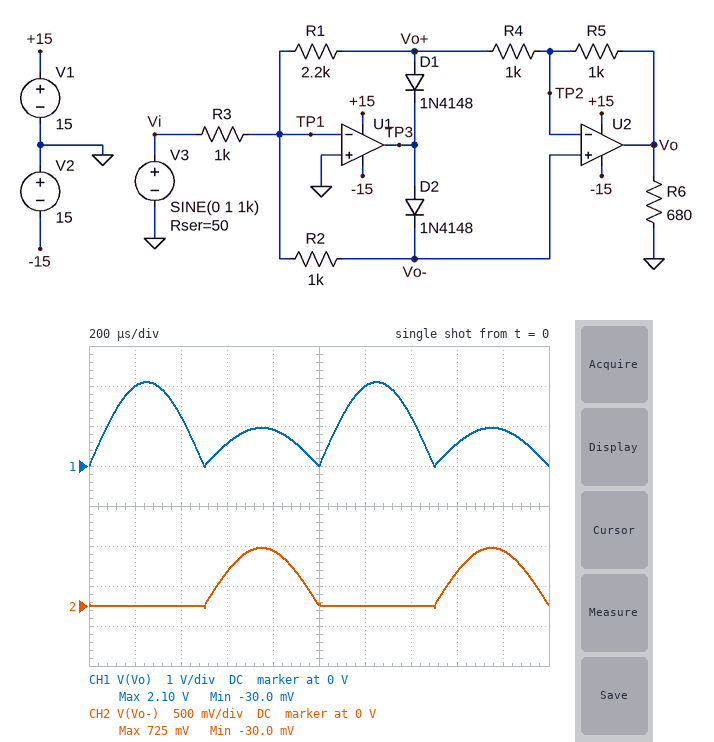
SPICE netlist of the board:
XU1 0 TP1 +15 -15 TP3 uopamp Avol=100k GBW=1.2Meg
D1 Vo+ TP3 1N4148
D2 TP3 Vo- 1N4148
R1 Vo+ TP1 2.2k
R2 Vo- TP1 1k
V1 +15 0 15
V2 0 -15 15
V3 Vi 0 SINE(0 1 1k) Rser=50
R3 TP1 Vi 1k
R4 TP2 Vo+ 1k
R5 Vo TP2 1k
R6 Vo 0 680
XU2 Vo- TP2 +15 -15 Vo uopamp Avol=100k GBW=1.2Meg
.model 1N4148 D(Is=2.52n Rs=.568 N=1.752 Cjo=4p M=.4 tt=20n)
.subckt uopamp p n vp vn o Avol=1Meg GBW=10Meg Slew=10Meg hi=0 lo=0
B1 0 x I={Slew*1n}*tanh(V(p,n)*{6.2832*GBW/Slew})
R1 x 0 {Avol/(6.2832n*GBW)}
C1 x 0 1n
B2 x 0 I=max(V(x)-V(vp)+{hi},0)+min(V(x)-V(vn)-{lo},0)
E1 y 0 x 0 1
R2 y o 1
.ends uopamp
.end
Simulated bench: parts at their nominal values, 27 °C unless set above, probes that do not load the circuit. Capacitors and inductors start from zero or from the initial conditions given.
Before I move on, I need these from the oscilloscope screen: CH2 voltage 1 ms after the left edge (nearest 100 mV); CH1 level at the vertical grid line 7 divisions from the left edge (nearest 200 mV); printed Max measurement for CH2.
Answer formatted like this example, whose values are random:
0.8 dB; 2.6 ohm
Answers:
0 V; 1.2 V; 725 mV
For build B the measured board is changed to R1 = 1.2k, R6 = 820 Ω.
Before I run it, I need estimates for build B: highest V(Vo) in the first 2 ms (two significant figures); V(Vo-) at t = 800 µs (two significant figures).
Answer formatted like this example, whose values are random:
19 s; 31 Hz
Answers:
1.1 V; 620 mV
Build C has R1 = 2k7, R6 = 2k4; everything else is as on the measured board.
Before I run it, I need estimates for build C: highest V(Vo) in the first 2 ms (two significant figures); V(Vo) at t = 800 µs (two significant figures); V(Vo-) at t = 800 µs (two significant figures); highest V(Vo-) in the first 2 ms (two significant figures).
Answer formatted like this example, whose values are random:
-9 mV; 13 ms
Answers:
2.6 V; 910 mV; 710 mV; 750 mV
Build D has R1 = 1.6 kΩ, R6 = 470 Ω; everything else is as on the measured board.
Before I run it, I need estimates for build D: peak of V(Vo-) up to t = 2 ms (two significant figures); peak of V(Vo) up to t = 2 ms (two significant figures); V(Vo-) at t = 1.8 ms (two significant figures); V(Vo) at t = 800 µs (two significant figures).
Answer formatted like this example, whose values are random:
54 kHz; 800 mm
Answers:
690 mV; 1.5 V; 650 mV; 910 mV
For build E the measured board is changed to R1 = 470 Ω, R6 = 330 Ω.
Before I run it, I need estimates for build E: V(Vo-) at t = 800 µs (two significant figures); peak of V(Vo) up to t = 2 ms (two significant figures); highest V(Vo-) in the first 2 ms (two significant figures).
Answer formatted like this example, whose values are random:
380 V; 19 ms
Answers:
540 mV; 950 mV; 570 mV
